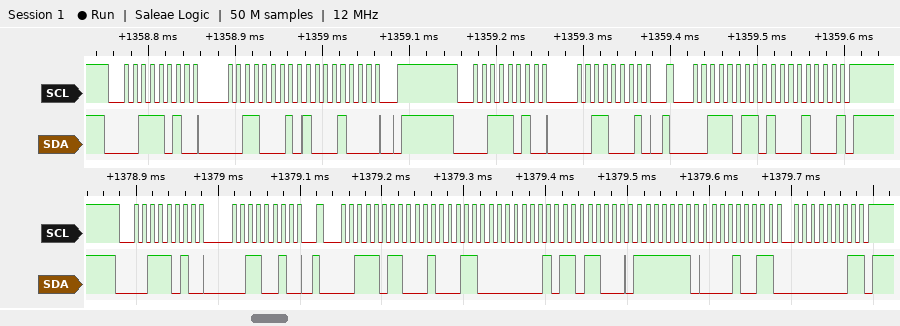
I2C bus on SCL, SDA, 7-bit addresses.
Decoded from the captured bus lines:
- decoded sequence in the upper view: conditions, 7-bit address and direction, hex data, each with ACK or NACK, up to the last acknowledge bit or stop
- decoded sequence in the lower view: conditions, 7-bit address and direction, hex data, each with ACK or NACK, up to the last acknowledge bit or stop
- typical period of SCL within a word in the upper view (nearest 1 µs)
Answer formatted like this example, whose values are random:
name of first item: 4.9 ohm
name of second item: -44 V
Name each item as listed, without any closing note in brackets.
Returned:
decoded sequence in the upper view: conditions, 7-bit address and direction, hex data, each with ACK or NACK, up to the last acknowledge bit or stop: start, address 1D write ACK, 31 ACK, 88 ACK, stop, start, address 1D write ACK, 31 ACK, repeated start, address 1D read ACK, 88 NACK, stop
decoded sequence in the lower view: conditions, 7-bit address and direction, hex data, each with ACK or NACK, up to the last acknowledge bit or stop: start, address 1D write ACK, 32 ACK, repeated start, address 1D read ACK, 23 ACK, 01 ACK, D8 ACK, FE ACK, 13 ACK, 01 NACK, stop
typical period of SCL within a word in the upper view: 10 µs
